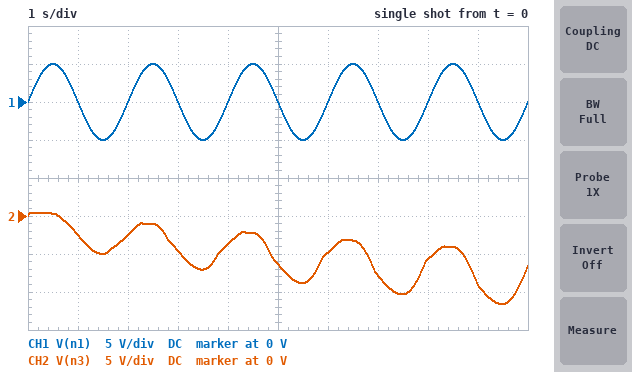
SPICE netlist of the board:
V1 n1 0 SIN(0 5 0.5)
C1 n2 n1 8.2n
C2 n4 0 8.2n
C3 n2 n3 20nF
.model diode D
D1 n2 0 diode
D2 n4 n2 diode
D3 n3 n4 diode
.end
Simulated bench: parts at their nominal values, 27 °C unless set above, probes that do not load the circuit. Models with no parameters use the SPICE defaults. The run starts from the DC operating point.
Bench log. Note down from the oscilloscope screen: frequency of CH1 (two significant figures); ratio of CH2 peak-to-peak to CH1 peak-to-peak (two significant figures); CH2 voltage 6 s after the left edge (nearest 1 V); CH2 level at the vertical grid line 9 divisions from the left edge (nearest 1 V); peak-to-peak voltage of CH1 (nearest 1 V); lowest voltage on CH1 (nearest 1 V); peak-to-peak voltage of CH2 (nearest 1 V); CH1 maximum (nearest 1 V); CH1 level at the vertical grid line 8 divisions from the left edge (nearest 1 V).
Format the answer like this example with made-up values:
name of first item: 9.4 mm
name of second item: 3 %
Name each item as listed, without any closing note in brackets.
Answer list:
frequency of CH1: 500 mHz
ratio of CH2 peak-to-peak to CH1 peak-to-peak: 1.2
CH2 voltage 6 s after the left edge: -5 V
CH2 level at the vertical grid line 9 divisions from the left edge: -9 V
peak-to-peak voltage of CH1: 10 V
lowest voltage on CH1: -5 V
peak-to-peak voltage of CH2: 12 V
CH1 maximum: 5 V
CH1 level at the vertical grid line 8 divisions from the left edge: 0 V
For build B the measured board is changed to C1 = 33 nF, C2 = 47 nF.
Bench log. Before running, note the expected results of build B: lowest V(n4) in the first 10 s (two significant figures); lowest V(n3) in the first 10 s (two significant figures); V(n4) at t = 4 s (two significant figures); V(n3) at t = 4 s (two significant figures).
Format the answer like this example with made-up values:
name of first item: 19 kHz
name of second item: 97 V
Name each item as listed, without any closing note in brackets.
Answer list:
lowest V(n4) in the first 10 s: -7.9 V
lowest V(n3) in the first 10 s: -15 V
V(n4) at t = 4 s: -5.1 V
V(n3) at t = 4 s: -4.7 V
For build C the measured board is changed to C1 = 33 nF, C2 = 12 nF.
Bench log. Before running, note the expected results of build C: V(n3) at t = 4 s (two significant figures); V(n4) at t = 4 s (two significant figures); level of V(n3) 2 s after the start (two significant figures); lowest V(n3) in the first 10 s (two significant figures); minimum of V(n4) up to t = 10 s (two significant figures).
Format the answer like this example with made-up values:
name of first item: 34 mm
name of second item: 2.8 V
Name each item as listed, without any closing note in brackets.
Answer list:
V(n3) at t = 4 s: -6.2 V
V(n4) at t = 4 s: -6.7 V
level of V(n3) 2 s after the start: -4.2 V
lowest V(n3) in the first 10 s: -16 V
minimum of V(n4) up to t = 10 s: -8.6 V
